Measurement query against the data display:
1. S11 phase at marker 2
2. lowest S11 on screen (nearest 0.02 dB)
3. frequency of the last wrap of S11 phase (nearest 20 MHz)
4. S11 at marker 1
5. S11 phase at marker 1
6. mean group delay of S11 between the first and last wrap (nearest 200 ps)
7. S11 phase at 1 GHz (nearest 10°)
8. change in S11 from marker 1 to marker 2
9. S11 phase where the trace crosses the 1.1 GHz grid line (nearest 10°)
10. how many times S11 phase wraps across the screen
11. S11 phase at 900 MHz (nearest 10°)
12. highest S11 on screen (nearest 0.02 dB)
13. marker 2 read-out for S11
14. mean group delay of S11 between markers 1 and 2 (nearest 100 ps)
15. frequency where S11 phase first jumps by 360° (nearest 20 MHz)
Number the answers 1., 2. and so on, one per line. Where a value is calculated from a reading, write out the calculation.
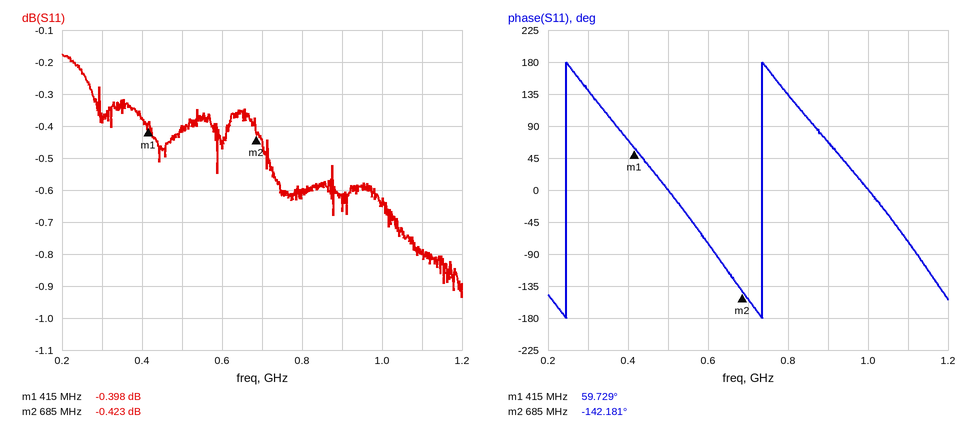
1. -142.181°
2. -0.94 dB
3. 740 MHz
4. -0.398 dB
5. 59.729°
6. 1 cycle / (740 MHz − 240 MHz) ≈ 2.0 ns
7. 0°
8. -0.423 − (-0.398) = -0.025 dB
9. -70°
10. 2
11. 70°
12. -0.18 dB
13. -0.423 dB
14. −(-142.181° − (59.729°))/(360° × 270 MHz) ≈ 2.1 ns
15. 240 MHz
